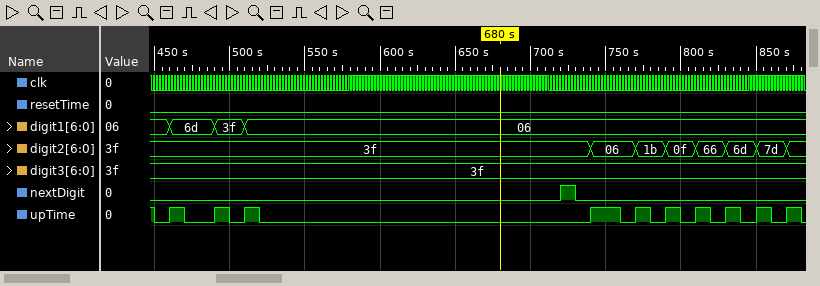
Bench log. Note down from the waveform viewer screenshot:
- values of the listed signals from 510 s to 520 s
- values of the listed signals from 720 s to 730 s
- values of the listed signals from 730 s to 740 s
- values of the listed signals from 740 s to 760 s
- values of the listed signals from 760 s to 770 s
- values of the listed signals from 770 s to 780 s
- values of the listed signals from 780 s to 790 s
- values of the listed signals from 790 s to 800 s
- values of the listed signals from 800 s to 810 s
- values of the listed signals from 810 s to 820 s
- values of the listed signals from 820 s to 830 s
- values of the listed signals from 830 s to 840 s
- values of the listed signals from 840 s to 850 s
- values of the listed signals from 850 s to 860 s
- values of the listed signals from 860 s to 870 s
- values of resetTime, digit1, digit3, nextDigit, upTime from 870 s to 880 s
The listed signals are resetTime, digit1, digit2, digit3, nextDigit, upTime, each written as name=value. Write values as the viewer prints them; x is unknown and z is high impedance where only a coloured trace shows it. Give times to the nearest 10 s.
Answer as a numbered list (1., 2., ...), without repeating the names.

1. resetTime=0, digit1=06, digit2=3f, digit3=3f, nextDigit=0, upTime=1
2. resetTime=0, digit1=06, digit2=3f, digit3=3f, nextDigit=1, upTime=0
3. resetTime=0, digit1=06, digit2=3f, digit3=3f, nextDigit=0, upTime=0
4. resetTime=0, digit1=06, digit2=06, digit3=3f, nextDigit=0, upTime=1
5. resetTime=0, digit1=06, digit2=06, digit3=3f, nextDigit=0, upTime=0
6. resetTime=0, digit1=06, digit2=1b, digit3=3f, nextDigit=0, upTime=1
7. resetTime=0, digit1=06, digit2=1b, digit3=3f, nextDigit=0, upTime=0
8. resetTime=0, digit1=06, digit2=0f, digit3=3f, nextDigit=0, upTime=1
9. resetTime=0, digit1=06, digit2=0f, digit3=3f, nextDigit=0, upTime=0
10. resetTime=0, digit1=06, digit2=66, digit3=3f, nextDigit=0, upTime=1
11. resetTime=0, digit1=06, digit2=66, digit3=3f, nextDigit=0, upTime=0
12. resetTime=0, digit1=06, digit2=6d, digit3=3f, nextDigit=0, upTime=1
13. resetTime=0, digit1=06, digit2=6d, digit3=3f, nextDigit=0, upTime=0
14. resetTime=0, digit1=06, digit2=7d, digit3=3f, nextDigit=0, upTime=1
15. resetTime=0, digit1=06, digit2=7d, digit3=3f, nextDigit=0, upTime=0
16. resetTime=0, digit1=06, digit3=3f, nextDigit=0, upTime=1
